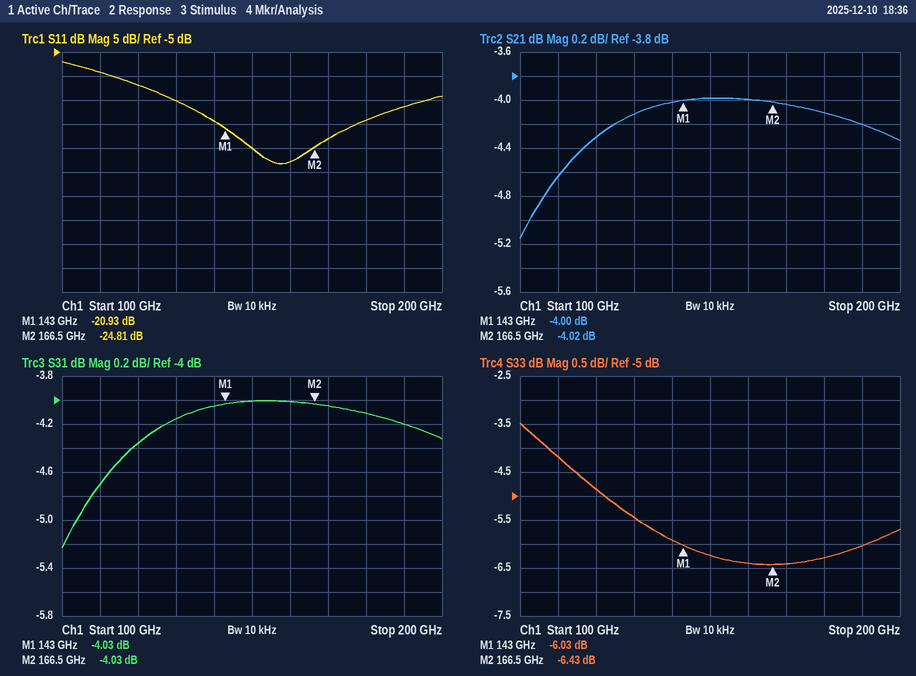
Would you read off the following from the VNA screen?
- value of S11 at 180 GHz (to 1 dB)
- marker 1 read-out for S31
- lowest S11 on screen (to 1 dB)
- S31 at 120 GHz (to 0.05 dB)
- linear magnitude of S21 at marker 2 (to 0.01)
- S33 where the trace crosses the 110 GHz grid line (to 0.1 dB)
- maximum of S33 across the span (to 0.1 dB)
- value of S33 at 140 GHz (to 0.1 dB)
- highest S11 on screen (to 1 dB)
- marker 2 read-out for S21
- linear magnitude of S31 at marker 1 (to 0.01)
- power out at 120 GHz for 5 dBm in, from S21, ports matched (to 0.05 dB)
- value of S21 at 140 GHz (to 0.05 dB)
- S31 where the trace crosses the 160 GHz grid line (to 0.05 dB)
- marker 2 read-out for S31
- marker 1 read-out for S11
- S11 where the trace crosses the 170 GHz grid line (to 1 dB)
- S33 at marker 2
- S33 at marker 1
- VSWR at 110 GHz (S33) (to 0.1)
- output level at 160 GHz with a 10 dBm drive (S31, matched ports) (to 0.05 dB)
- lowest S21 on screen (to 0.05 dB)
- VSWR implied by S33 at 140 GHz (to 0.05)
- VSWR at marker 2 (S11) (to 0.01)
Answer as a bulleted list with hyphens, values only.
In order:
- -19 dB
- -4.03 dB
- -28 dB
- -4.35 dB
- 0.63
- -4.2 dB
- -3.5 dB
- -5.9 dB
- -7 dB
- -4.02 dB
- 0.63
- 0.70 dBm
- -4.00 dB
- -4.00 dB
- -4.03 dB
- -20.93 dB
- -23 dB
- -6.43 dB
- -6.03 dB
- 4.2
- 6.00 dBm
- -5.15 dB
- 3.05
- 1.12
